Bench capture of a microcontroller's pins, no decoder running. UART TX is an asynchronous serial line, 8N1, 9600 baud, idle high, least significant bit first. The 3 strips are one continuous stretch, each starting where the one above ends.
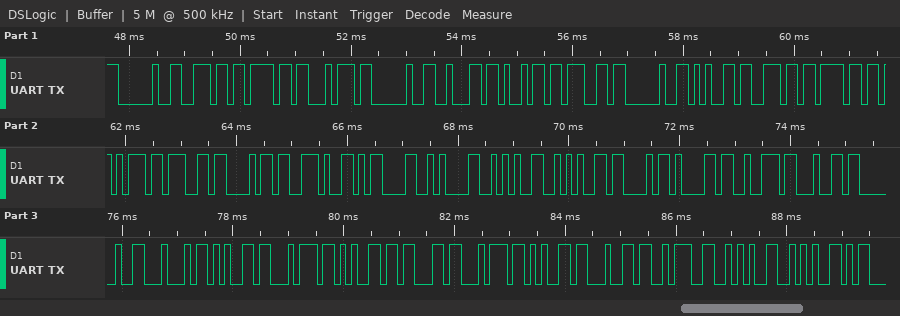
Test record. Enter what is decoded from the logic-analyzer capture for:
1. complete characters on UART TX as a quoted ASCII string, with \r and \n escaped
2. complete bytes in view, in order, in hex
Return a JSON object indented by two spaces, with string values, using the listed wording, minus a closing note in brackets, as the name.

{
  "complete characters on UART TX as a quoted ASCII string, with \\r and \\n escaped": "\" not big enough.\\r\\n**Card Detected:**\"",
  "complete bytes in view, in order, in hex": "20 6E 6F 74 20 62 69 67 20 65 6E 6F 75 67 68 2E 0D 0A 2A 2A 43 61 72 64 20 44 65 74 65 63 74 65 64 3A 2A 2A"
}
